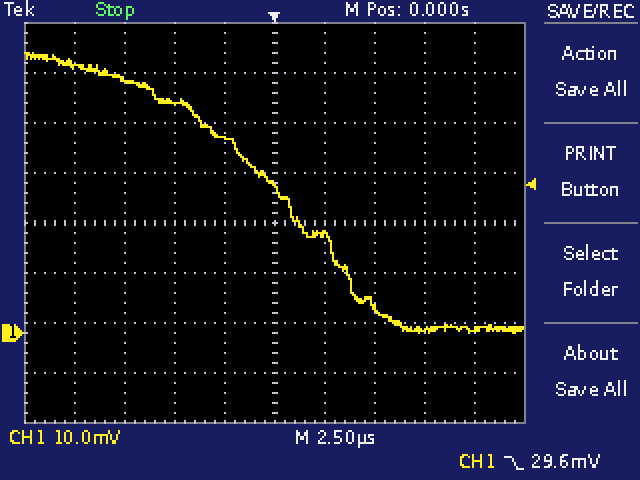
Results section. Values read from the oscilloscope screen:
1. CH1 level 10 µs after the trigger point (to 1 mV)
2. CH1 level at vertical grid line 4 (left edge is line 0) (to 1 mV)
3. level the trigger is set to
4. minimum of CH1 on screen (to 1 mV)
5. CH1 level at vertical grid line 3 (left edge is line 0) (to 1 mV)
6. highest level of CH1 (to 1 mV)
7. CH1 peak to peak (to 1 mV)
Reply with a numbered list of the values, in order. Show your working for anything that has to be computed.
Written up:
1. 1 mV
2. 39 mV
3. 29.6 mV
4. 0 mV
5. 46 mV
6. 56 mV
7. 56 mV − (0 mV) = 56 mV
